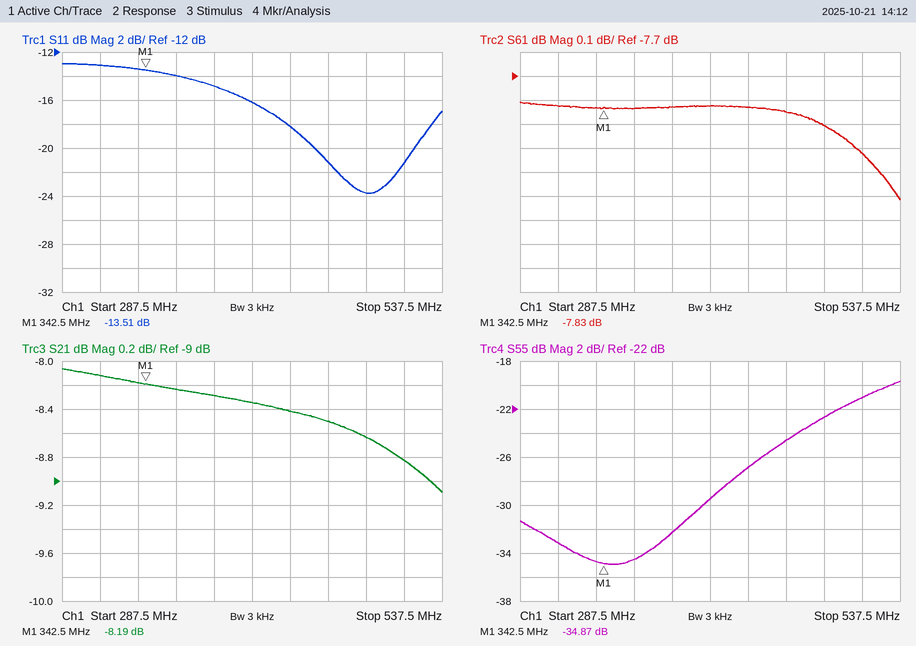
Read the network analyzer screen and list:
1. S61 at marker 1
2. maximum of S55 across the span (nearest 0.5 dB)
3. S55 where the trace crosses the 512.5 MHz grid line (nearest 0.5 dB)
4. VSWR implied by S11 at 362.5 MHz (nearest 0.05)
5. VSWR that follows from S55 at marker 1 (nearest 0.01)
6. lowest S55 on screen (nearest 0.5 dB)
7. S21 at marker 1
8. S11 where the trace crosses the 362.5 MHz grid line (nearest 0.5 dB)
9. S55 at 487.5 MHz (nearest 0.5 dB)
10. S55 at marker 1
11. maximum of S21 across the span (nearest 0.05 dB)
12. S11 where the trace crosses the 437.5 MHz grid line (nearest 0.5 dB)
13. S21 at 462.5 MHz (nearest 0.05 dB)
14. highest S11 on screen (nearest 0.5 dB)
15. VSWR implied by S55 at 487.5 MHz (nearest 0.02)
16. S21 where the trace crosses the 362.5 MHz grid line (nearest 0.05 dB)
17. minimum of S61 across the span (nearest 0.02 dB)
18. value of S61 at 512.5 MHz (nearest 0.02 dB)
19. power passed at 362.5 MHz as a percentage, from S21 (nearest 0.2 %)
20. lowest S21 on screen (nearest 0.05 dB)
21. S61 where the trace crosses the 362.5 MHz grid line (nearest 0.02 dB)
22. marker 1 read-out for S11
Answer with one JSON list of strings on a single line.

["-7.83 dB", "-19.5 dB", "-21.0 dB", "1.50", "1.04", "-35.0 dB", "-8.19 dB", "-14.0 dB", "-22.5 dB", "-34.87 dB", "-8.05 dB", "-18.0 dB", "-8.50 dB", "-13.0 dB", "1.16", "-8.25 dB", "-8.22 dB", "-8.02 dB", "15.0 %", "-9.10 dB", "-7.84 dB", "-13.51 dB"]
